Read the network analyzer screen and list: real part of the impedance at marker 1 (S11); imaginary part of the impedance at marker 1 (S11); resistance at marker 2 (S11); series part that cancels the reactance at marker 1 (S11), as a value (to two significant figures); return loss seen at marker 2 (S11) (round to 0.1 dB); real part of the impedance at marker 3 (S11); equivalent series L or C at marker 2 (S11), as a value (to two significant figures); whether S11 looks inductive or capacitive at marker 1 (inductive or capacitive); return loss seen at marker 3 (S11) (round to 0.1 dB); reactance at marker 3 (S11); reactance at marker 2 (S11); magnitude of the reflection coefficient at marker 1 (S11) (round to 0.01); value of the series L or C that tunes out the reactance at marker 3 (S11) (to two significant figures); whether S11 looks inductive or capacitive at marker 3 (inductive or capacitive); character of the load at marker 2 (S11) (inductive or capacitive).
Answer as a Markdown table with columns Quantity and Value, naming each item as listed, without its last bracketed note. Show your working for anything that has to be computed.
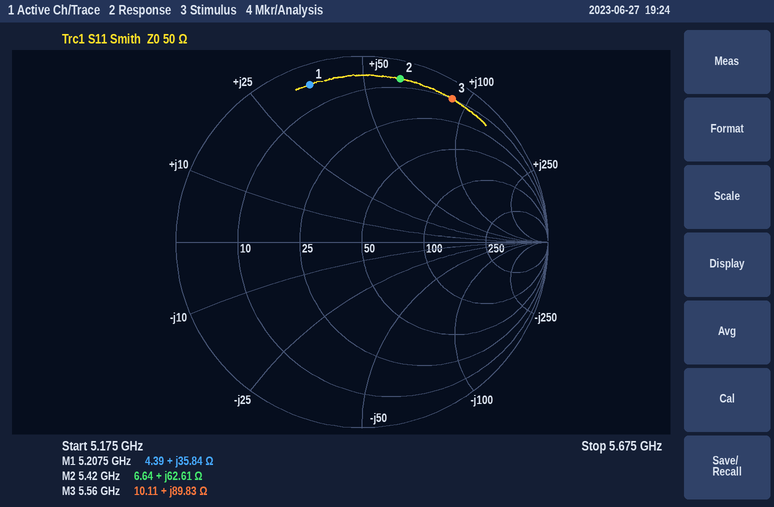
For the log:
| Quantity | Value |
|---|---|
| real part of the impedance at marker 1 | 4.39 Ω |
| imaginary part of the impedance at marker 1 | +35.84 Ω |
| resistance at marker 2 | 6.64 Ω |
| series part that cancels the reactance at marker 1 (S11), as a value | C = 1/(2π × 5.2075 GHz × 35.84 Ω) ≈ 853 fF, so 850 fF to two significant figures |
| return loss seen at marker 2 (S11) | 0.9 dB |
| real part of the impedance at marker 3 | 10.11 Ω |
| equivalent series L or C at marker 2 (S11), as a value | L = 62.61 Ω/(2π × 5.42 GHz) ≈ 1.8 nH |
| whether S11 looks inductive or capacitive at marker 1 | inductive |
| return loss seen at marker 3 (S11) | 0.8 dB |
| reactance at marker 3 | +89.83 Ω |
| reactance at marker 2 | +62.61 Ω |
| magnitude of the reflection coefficient at marker 1 (S11) | 0.89 |
| value of the series L or C that tunes out the reactance at marker 3 (S11) | C = 1/(2π × 5.56 GHz × 89.83 Ω) ≈ 319 fF, so 320 fF to two significant figures |
| whether S11 looks inductive or capacitive at marker 3 | inductive |
| character of the load at marker 2 (S11) | inductive |
